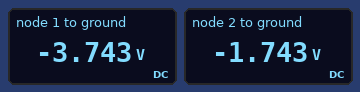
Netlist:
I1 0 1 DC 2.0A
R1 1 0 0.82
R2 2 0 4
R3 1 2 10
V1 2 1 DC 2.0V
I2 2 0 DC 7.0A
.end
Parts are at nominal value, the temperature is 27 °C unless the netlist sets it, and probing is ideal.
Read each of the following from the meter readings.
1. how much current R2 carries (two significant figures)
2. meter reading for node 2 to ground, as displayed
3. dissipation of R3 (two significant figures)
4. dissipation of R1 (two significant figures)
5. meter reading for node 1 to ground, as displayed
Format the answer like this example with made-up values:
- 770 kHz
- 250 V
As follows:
- 440 mA
- -1.743 V
- 400 mW
- 17 W
- -3.743 V
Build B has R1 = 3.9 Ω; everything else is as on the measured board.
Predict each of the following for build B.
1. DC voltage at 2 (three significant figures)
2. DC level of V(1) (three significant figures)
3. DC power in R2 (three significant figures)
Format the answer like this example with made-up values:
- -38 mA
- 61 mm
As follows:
- -8.86 V
- -10.9 V
- 19.6 W
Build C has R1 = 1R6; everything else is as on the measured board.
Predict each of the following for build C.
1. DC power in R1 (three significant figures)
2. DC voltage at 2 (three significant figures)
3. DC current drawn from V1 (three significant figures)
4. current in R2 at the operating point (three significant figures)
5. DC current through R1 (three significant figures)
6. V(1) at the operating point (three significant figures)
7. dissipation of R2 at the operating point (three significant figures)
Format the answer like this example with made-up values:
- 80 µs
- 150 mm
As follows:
- 24.7 W
- -4.29 V
- 6.13 A
- 1.07 A
- 3.93 A
- -6.29 V
- 4.59 W
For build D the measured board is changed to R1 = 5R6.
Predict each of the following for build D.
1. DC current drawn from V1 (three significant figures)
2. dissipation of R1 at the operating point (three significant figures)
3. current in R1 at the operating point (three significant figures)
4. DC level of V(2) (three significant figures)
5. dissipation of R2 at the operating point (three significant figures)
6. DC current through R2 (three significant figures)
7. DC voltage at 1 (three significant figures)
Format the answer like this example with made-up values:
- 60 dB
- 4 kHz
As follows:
- 4.49 A
- 29.4 W
- 2.29 A
- -10.8 V
- 29.3 W
- 2.71 A
- -12.8 V
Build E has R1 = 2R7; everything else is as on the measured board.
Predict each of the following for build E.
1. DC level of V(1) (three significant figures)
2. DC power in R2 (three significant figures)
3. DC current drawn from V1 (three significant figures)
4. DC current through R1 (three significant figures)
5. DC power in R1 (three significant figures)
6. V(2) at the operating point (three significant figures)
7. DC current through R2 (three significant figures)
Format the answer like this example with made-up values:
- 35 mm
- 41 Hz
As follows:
- -8.87 V
- 11.8 W
- 5.48 A
- 3.28 A
- 29.1 W
- -6.87 V
- 1.72 A
